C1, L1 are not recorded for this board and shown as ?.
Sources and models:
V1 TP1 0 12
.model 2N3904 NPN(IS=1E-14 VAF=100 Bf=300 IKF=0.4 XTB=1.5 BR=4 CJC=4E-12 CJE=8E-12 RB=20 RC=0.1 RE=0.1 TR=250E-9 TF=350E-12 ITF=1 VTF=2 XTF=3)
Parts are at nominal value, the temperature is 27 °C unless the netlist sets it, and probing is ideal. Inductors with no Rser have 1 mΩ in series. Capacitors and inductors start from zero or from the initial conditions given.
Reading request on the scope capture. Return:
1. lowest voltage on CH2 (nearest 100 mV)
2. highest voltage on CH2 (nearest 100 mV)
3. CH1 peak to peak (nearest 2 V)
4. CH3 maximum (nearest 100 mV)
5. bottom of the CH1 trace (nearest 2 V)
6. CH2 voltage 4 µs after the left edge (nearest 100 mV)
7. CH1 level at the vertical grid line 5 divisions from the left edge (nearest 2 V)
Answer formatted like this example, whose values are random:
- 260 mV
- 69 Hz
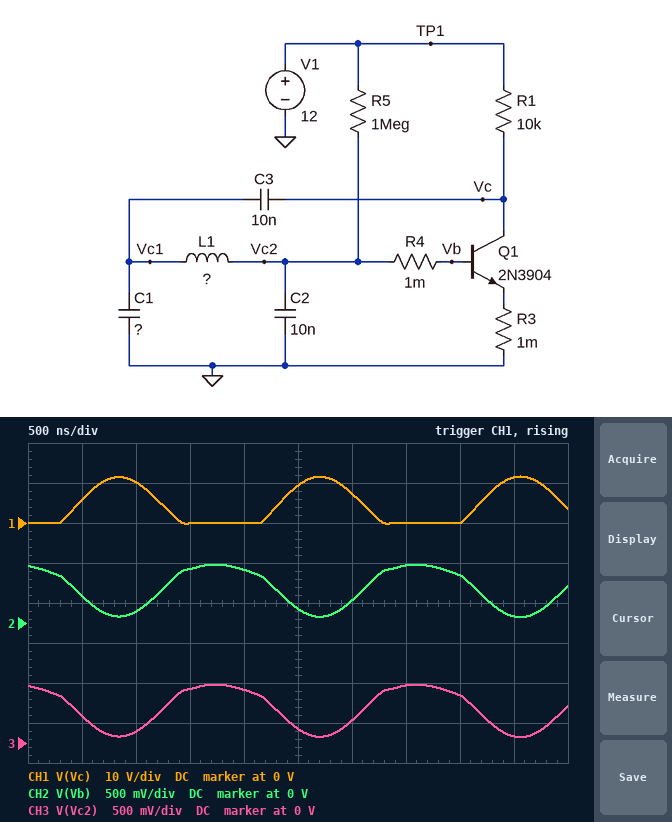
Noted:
- 100 mV
- 700 mV
- 12 V
- 700 mV
- 0 V
- 600 mV
- 10 V
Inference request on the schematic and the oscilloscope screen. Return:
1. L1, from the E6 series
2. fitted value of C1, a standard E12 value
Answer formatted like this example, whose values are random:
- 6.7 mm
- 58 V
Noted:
- 150 µH
- 470 pF
